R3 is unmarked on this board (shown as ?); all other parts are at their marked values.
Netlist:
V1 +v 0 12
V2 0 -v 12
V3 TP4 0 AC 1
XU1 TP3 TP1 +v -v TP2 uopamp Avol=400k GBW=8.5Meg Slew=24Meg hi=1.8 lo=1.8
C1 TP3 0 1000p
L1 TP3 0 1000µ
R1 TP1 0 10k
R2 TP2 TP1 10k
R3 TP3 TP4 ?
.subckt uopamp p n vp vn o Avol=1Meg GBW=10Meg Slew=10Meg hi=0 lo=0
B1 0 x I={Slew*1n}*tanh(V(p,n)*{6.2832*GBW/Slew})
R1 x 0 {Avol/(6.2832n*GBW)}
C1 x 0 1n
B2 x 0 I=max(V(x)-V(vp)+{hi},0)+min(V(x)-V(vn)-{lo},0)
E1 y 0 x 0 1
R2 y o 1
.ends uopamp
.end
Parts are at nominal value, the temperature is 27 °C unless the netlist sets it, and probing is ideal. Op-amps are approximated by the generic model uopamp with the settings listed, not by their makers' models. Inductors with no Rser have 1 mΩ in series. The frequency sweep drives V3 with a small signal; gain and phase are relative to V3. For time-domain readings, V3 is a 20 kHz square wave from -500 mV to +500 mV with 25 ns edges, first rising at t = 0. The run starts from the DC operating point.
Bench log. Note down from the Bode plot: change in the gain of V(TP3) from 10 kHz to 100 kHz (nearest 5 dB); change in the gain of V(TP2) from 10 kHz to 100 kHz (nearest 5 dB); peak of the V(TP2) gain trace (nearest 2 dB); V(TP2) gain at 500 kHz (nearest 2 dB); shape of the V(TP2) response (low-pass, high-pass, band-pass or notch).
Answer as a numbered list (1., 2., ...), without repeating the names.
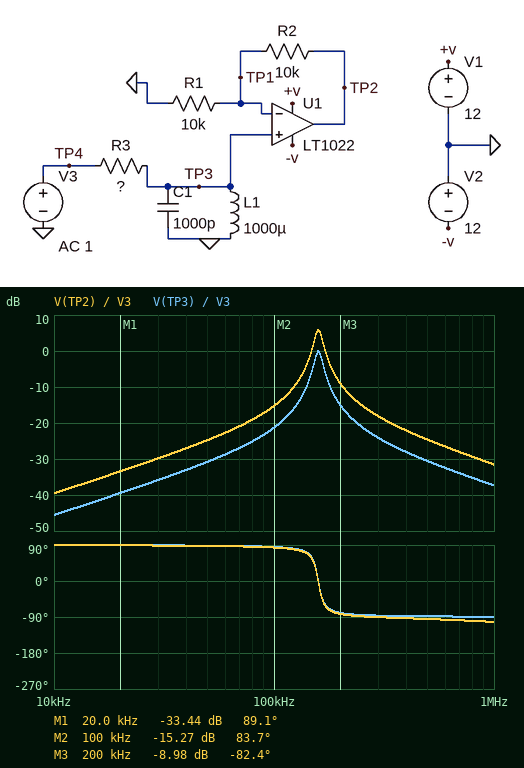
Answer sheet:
1. 25 dB
2. 25 dB
3. 6 dB
4. -24 dB
5. band-pass
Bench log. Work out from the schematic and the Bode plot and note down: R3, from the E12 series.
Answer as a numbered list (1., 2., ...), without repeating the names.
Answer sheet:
1. 12 kΩ
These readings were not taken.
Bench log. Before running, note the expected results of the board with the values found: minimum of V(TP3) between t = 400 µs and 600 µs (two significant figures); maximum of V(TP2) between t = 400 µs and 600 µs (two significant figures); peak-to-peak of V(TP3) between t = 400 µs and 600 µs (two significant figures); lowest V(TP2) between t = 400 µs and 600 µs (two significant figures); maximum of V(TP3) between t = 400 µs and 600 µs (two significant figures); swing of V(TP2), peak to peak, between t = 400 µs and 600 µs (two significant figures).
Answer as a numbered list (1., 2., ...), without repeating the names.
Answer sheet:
1. -58 mV
2. 120 mV
3. 120 mV
4. -120 mV
5. 58 mV
6. 230 mV
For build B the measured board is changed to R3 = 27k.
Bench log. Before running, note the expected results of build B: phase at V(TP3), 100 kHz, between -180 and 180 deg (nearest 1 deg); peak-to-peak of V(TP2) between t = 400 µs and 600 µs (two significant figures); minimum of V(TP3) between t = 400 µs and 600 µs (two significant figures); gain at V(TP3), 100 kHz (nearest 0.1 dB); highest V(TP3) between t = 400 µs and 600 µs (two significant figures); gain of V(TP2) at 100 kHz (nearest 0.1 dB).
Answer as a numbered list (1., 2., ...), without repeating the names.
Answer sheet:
1. 88 deg
2. 89 mV
3. -22 mV
4. -28.3 dB
5. 22 mV
6. -22.3 dB
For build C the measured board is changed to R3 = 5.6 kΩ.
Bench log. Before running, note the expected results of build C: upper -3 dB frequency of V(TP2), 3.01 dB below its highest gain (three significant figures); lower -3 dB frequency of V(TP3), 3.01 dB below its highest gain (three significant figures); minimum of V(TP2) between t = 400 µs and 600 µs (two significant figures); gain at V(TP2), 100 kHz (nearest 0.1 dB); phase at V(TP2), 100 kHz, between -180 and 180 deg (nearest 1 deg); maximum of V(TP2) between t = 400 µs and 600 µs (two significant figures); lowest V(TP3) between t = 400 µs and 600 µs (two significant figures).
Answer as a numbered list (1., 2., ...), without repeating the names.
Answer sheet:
1. 174 kHz
2. 146 kHz
3. -280 mV
4. -8.8 dB
5. 78 deg
6. 280 mV
7. -140 mV
